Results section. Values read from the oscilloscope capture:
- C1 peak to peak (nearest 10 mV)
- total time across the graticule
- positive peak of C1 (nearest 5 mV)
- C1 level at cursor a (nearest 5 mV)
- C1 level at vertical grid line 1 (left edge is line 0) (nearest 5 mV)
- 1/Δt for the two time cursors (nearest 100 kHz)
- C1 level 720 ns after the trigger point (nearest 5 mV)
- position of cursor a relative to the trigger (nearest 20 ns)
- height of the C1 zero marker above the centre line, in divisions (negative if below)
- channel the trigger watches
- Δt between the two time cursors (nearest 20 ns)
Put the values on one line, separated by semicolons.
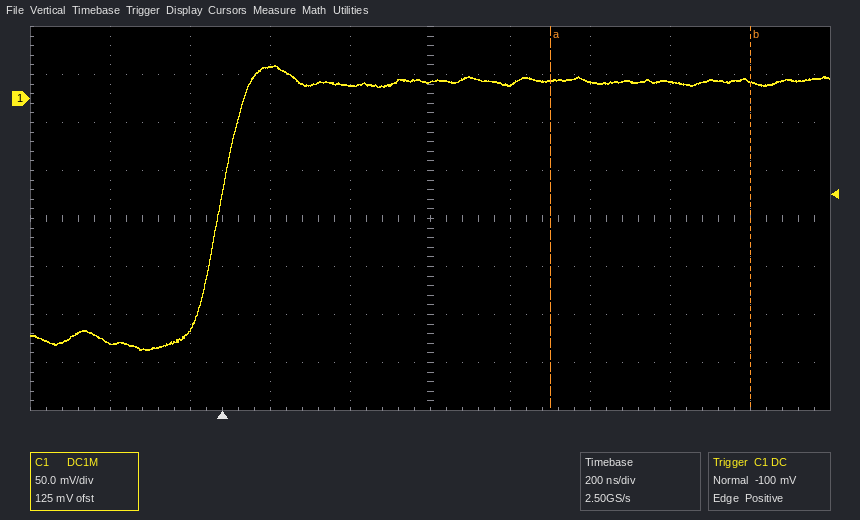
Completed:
300 mV; 2 µs; 35 mV; 20 mV; -255 mV; 2.0 MHz; 15 mV; +820 ns; +2.5 div; C1; 500 ns
